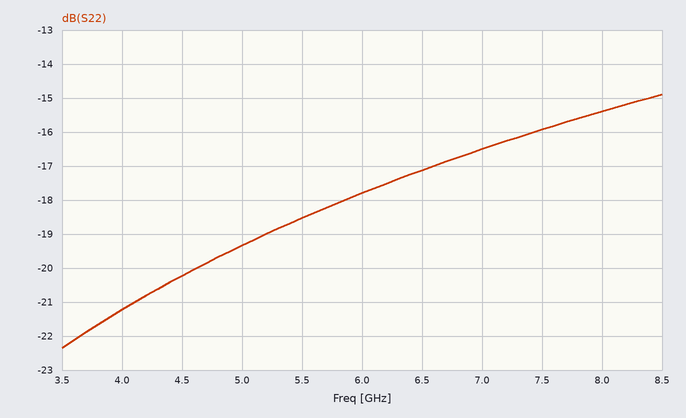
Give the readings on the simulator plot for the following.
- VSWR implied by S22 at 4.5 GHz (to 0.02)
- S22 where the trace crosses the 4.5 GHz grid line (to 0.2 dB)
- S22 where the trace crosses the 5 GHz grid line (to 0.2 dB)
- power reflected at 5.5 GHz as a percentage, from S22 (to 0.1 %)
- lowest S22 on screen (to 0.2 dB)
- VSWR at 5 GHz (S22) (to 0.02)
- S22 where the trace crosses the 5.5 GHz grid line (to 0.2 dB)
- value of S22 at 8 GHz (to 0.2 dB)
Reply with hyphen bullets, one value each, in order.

- 1.22
- -20.2 dB
- -19.4 dB
- 1.4 %
- -22.4 dB
- 1.24
- -18.6 dB
- -15.4 dB
